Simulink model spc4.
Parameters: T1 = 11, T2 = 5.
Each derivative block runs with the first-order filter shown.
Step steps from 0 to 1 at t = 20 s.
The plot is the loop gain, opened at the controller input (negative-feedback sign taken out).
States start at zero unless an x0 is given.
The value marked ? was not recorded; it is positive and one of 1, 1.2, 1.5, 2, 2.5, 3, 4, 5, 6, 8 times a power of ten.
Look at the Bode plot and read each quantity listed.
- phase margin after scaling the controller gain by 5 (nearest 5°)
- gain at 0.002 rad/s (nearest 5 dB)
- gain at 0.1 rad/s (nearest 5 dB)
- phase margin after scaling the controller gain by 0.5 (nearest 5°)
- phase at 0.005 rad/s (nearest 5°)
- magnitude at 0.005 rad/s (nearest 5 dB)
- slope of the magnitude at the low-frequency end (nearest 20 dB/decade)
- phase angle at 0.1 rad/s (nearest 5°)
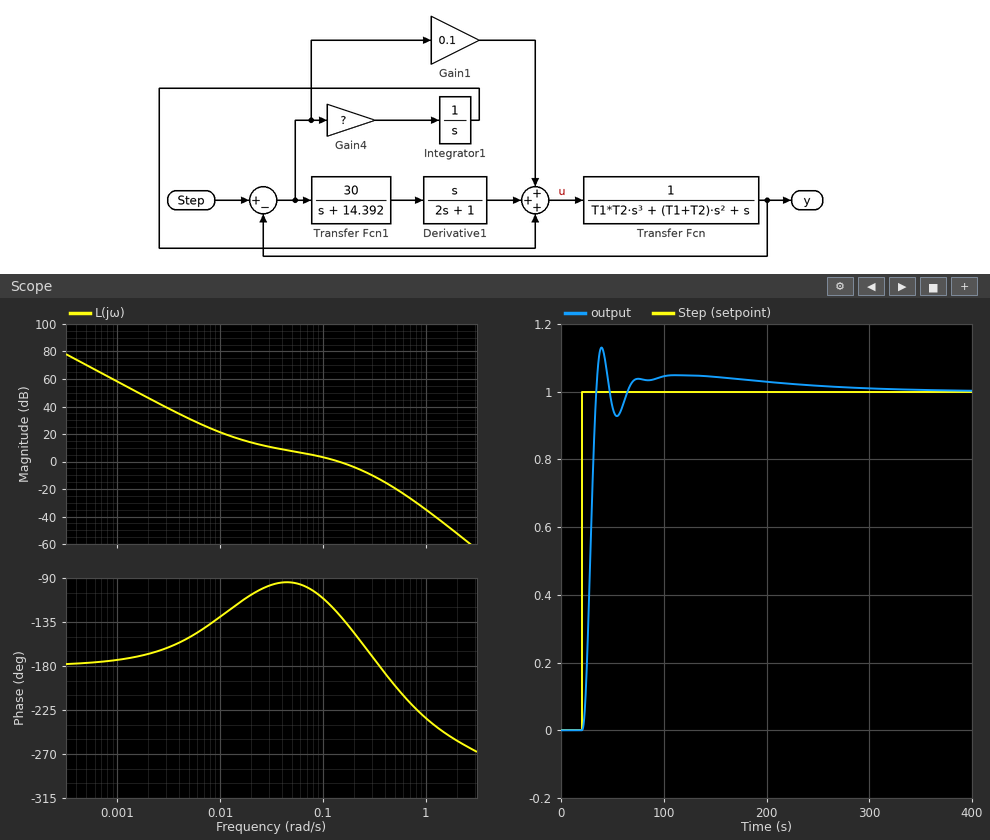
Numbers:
-5°
45 dB
5 dB
80°
-150°
30 dB
-40 dB/decade
-110°
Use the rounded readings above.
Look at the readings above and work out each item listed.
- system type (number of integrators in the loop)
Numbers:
2
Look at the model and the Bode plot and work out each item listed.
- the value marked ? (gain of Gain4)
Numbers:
0.0008
